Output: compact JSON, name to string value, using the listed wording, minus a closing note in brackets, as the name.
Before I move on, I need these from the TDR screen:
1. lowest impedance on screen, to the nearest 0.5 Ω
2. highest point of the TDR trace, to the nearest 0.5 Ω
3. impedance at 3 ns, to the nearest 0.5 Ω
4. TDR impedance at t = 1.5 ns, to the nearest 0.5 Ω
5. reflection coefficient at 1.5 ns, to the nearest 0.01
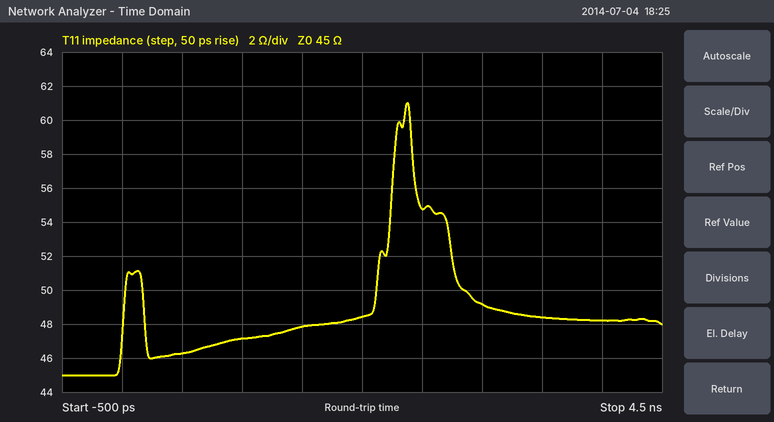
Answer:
{"lowest impedance on screen, to the nearest 0.5 Ω": "45.0 Ω", "highest point of the TDR trace, to the nearest 0.5 Ω": "61.0 Ω", "impedance at 3 ns, to the nearest 0.5 Ω": "49.0 Ω", "TDR impedance at t = 1.5 ns, to the nearest 0.5 Ω": "48.0 Ω", "reflection coefficient at 1.5 ns, to the nearest 0.01": "+0.03"}
